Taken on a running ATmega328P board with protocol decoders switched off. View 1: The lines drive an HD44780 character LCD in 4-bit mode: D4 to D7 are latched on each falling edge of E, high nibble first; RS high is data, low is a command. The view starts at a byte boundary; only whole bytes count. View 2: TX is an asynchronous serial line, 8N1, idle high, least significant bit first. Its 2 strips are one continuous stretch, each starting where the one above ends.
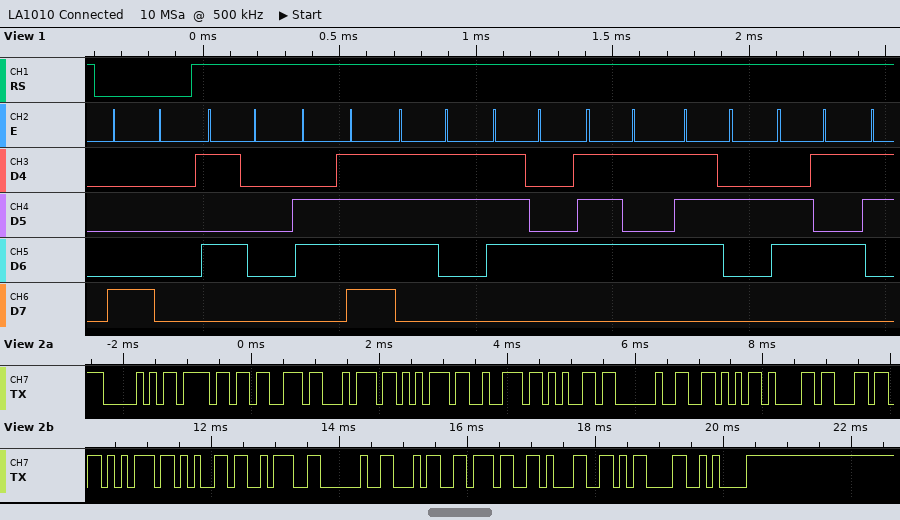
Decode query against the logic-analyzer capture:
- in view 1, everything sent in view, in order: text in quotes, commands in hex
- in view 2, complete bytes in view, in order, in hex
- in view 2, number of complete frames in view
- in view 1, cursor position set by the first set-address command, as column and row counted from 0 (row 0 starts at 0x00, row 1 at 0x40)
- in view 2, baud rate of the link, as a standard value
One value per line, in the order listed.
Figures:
0x80 "Posture"
0x50 0x6F 0x73 0x74 0x75 0x72 0x65 0x20 0x56 0x61 0x6C 0x75 0x65 0x3A 0x20 0x34 0x37 0x31 0x0D 0x0A
20
column 0, row 0
9600 baud
